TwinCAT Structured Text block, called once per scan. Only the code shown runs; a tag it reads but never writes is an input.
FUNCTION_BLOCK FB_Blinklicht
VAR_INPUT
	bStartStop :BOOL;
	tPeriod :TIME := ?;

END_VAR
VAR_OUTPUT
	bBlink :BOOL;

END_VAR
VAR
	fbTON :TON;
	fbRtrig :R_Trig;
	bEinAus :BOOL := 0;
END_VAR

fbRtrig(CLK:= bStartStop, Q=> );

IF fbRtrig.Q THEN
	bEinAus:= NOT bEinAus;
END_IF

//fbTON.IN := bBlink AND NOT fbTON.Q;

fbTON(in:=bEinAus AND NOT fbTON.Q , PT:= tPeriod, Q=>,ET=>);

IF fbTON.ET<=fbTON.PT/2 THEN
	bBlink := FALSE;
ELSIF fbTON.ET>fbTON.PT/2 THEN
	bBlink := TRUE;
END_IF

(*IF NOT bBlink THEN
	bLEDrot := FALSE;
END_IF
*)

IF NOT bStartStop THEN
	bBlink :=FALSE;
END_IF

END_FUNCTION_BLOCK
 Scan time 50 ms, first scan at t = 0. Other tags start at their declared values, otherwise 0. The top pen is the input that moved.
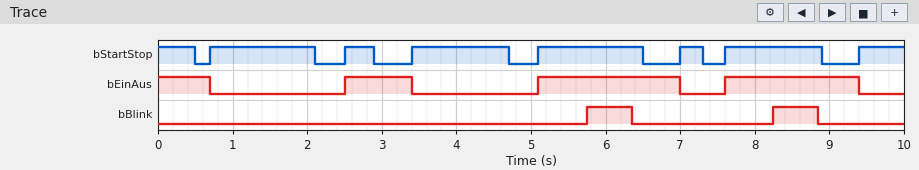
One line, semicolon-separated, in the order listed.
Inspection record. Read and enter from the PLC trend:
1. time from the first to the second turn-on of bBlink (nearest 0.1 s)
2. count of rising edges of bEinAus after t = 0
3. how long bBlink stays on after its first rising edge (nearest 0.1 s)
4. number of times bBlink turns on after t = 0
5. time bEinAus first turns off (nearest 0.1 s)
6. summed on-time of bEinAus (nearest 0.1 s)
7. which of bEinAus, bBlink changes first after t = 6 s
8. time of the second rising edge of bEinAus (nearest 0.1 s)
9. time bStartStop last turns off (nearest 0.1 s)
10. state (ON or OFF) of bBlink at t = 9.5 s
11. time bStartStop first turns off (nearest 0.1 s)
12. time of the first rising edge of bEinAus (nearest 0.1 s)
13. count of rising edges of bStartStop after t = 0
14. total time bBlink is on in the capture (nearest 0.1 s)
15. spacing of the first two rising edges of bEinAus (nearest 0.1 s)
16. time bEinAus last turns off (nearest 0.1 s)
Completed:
2.5 s; 3; 0.6 s; 2; 0.7 s; 5.3 s; bBlink; 5.1 s; 8.9 s; OFF; 0.5 s; 2.5 s; 7; 1.2 s; 2.6 s; 9.4 s
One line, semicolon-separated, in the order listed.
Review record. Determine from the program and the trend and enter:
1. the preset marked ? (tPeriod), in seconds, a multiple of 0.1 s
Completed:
1.2 s
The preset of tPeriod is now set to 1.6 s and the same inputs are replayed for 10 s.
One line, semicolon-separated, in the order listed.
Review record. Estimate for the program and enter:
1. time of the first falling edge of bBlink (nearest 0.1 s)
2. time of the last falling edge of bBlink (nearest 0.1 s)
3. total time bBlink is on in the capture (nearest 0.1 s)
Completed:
6.5 s; 8.9 s; 1.0 s
